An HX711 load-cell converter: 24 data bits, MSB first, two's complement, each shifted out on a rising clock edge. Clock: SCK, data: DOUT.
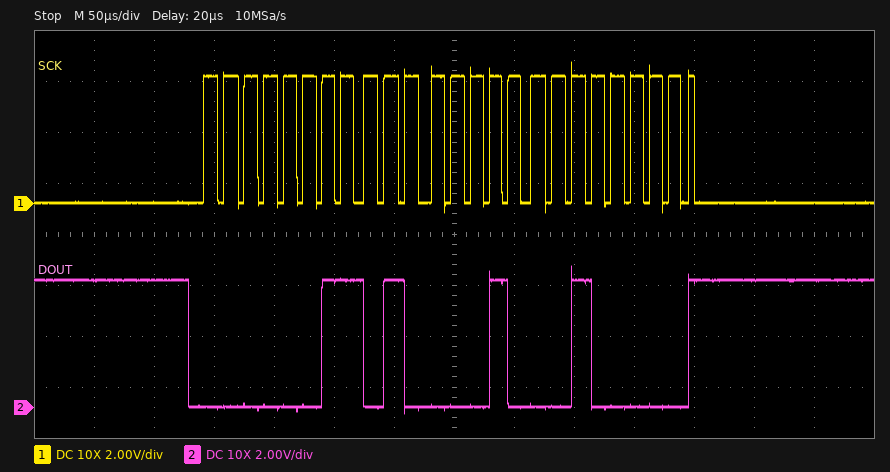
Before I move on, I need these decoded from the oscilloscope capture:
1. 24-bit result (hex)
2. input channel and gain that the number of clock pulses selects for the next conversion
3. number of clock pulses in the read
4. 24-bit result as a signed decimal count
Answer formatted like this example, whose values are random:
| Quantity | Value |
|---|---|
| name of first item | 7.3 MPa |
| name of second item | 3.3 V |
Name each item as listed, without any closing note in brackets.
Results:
| Quantity | Value |
|---|---|
| 24-bit result | 0x034220 |
| input channel and gain that the number of clock pulses selects for the next conversion | channel A, gain 128 |
| number of clock pulses in the read | 25 |
| 24-bit result as a signed decimal count | 213536 |
